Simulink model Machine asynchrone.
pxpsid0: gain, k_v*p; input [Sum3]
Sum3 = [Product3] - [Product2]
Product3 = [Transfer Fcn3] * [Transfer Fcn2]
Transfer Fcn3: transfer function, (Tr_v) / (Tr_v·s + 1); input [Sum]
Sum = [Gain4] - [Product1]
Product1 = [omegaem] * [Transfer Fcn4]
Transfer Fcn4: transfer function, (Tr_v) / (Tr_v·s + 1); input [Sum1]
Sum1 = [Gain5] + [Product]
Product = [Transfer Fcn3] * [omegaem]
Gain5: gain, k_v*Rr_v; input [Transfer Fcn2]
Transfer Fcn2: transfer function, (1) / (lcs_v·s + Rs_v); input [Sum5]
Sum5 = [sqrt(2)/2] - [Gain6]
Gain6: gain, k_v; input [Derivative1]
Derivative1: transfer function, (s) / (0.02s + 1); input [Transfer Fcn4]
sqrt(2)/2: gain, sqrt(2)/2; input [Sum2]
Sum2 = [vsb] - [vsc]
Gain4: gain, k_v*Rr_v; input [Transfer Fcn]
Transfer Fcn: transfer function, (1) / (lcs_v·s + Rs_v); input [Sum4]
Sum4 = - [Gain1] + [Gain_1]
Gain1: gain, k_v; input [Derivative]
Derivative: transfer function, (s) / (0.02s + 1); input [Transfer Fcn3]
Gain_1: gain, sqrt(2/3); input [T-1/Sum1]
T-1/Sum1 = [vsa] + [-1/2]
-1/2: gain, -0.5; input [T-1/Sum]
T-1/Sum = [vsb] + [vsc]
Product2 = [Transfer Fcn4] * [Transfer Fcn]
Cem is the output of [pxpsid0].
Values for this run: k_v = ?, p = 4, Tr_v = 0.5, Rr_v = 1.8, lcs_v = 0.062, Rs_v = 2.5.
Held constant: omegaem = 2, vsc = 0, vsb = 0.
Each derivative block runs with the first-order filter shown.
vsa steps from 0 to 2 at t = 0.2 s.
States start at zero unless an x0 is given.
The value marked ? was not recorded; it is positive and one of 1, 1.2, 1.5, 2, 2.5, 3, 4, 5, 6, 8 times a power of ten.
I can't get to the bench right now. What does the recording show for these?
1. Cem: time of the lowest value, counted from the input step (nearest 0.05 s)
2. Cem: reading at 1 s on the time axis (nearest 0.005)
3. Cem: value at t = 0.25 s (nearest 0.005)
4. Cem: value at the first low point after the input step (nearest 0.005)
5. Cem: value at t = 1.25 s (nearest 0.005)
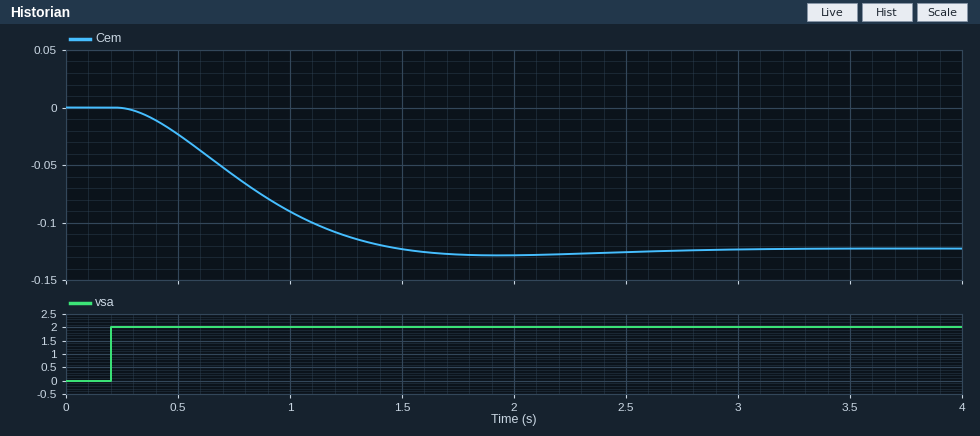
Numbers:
1.75 s
-0.090
0.000
-0.130
-0.110
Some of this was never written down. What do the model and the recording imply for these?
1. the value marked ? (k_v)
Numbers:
0.4
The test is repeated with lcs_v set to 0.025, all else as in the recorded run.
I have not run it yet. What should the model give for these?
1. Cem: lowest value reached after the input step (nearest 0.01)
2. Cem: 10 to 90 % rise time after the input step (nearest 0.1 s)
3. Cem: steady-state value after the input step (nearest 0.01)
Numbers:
-0.13
0.8 s
-0.12
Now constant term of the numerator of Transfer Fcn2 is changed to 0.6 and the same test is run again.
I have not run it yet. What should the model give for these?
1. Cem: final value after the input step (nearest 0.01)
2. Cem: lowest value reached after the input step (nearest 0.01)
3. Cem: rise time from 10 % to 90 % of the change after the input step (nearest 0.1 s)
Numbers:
-0.12
-0.13
0.8 s
